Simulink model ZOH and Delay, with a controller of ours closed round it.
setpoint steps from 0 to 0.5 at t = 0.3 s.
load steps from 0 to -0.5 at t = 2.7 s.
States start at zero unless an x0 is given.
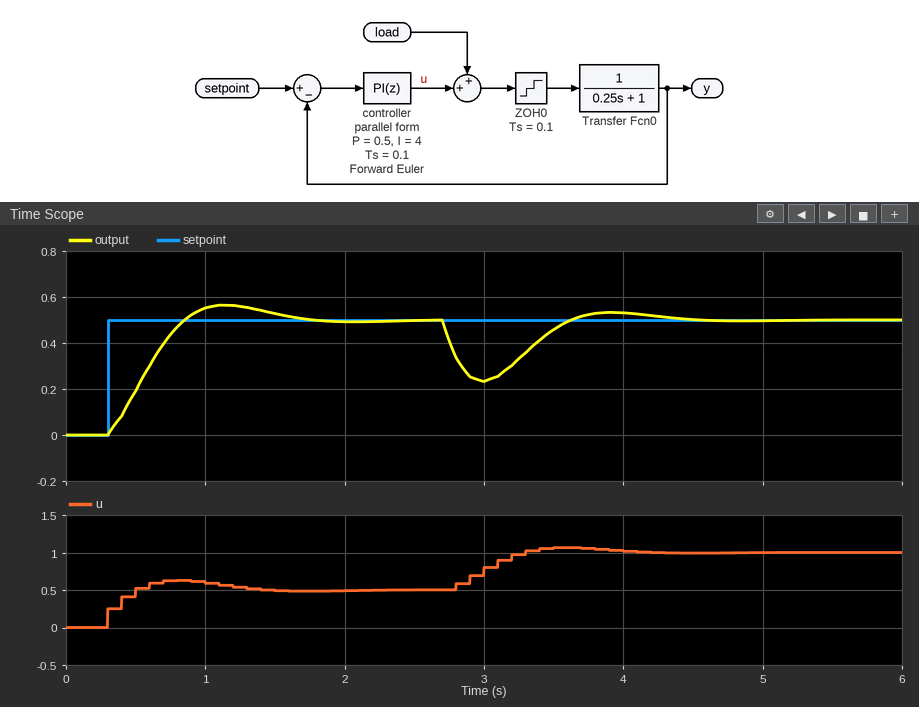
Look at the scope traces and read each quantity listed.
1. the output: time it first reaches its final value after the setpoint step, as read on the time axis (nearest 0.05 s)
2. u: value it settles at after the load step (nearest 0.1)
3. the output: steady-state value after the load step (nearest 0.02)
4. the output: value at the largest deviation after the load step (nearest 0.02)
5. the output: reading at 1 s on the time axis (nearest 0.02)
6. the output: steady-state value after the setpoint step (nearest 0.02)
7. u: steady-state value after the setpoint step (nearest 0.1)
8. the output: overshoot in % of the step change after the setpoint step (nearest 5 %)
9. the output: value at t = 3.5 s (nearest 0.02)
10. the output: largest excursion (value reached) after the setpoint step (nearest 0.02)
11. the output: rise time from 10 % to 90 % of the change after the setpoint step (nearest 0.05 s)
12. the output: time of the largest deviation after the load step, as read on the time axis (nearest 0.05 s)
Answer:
0.85 s
1.0
0.50
0.24
0.56
0.50
0.5
15 %
0.46
0.56
0.40 s
3.00 s
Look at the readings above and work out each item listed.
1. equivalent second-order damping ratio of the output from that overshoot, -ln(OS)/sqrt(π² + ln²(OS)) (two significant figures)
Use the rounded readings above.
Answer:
0.52
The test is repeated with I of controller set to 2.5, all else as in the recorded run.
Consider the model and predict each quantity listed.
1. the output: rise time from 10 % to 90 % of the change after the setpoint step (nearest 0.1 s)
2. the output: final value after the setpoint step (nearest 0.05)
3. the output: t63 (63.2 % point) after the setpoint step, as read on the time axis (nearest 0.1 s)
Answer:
0.7 s
0.50
0.7 s
